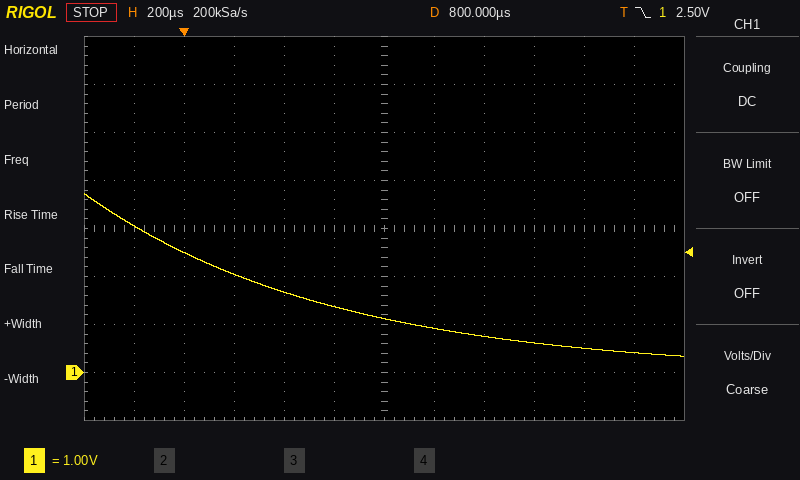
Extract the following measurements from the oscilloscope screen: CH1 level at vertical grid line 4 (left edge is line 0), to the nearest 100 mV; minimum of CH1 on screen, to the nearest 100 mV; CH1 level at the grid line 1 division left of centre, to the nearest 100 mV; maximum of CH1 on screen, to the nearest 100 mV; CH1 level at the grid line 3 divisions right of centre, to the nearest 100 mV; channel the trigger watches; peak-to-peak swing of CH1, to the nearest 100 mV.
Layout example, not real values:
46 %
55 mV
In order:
1.7 V
300 mV
1.4 V
3.7 V
600 mV
CH1
3.4 V
